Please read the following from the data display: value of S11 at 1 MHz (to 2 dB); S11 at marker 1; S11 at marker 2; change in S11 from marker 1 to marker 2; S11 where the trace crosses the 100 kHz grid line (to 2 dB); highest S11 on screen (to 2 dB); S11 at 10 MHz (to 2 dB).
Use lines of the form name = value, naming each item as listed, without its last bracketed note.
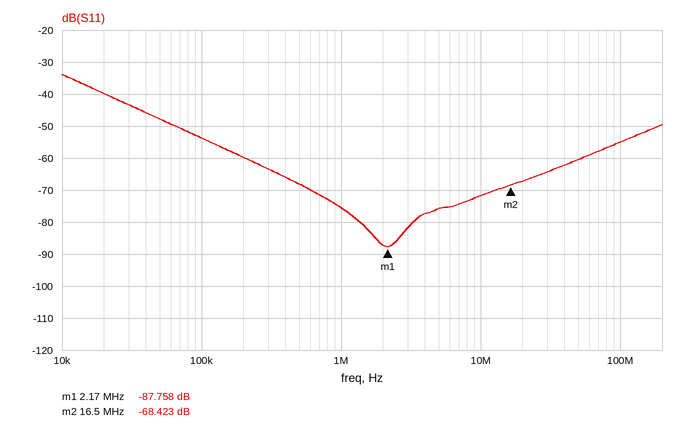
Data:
value of S11 at 1 MHz = -76 dB
S11 at marker 1 = -87.758 dB
S11 at marker 2 = -68.423 dB
change in S11 from marker 1 to marker 2 = 19.335 dB
S11 where the trace crosses the 100 kHz grid line = -54 dB
highest S11 on screen = -34 dB
S11 at 10 MHz = -72 dB
